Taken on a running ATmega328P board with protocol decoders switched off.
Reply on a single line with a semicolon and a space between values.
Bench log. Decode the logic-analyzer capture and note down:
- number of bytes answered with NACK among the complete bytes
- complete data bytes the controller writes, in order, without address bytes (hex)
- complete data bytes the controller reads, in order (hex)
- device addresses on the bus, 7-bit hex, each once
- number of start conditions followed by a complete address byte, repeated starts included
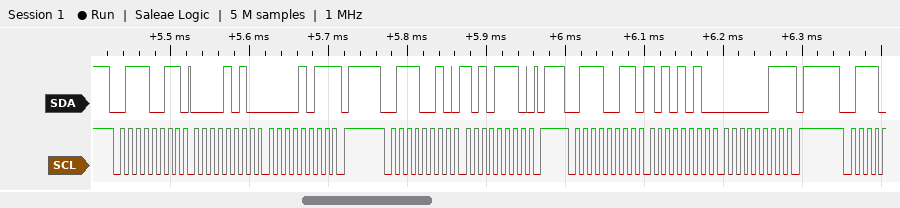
2; AE; 0A 0B AA 03; 0x39; 3
